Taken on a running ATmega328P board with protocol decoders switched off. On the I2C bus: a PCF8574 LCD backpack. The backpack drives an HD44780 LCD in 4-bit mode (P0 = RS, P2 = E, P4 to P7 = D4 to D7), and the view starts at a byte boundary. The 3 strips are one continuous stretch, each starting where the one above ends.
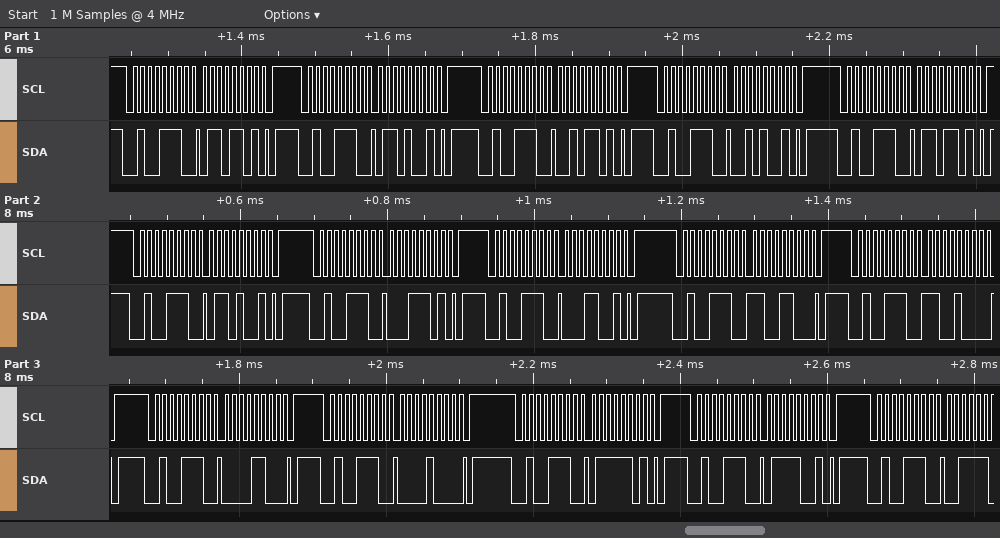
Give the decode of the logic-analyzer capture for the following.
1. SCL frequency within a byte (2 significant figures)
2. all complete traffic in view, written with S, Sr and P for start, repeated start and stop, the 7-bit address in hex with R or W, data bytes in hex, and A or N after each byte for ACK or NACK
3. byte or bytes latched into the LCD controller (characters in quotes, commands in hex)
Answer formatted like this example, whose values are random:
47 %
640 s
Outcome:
100 kHz
S 27W A 6D A P S 27W A 69 A P S 27W A 2D A P S 27W A 29 A P S 27W A 6D A P S 27W A 69 A P S 27W A 1D A P S 27W A 19 A P S 27W A CC A P S 27W A C8 A P S 27W A 0C A P S 27W A 08 A P S 27W A 7D A P S 27W A 79 A P S 27W A
'b' 'a' 0xC0
